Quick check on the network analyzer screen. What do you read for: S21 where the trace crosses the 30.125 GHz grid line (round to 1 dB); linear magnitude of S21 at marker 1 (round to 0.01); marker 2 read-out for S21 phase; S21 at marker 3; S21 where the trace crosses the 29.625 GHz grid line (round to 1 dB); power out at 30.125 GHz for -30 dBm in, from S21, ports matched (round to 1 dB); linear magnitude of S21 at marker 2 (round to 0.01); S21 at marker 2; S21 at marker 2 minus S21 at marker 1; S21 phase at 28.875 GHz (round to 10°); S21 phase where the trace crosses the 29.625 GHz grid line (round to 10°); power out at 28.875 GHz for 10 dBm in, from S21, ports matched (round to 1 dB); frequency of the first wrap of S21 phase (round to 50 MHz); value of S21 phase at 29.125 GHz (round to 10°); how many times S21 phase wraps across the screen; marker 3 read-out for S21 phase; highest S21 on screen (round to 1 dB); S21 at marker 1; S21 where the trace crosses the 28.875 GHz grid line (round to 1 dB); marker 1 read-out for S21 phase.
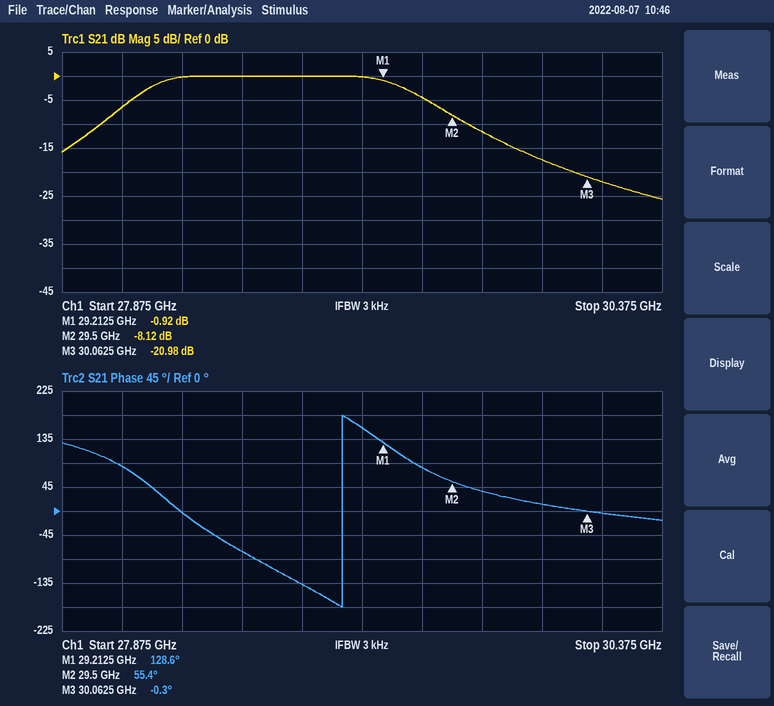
-22 dB
0.90
55.4°
-20.98 dB
-12 dB
-52 dBm
0.39
-8.12 dB
-7.20 dB
-140°
40°
10 dBm
29.05 GHz
160°
1
-0.3°
0 dB
-0.92 dB
0 dB
128.6°
